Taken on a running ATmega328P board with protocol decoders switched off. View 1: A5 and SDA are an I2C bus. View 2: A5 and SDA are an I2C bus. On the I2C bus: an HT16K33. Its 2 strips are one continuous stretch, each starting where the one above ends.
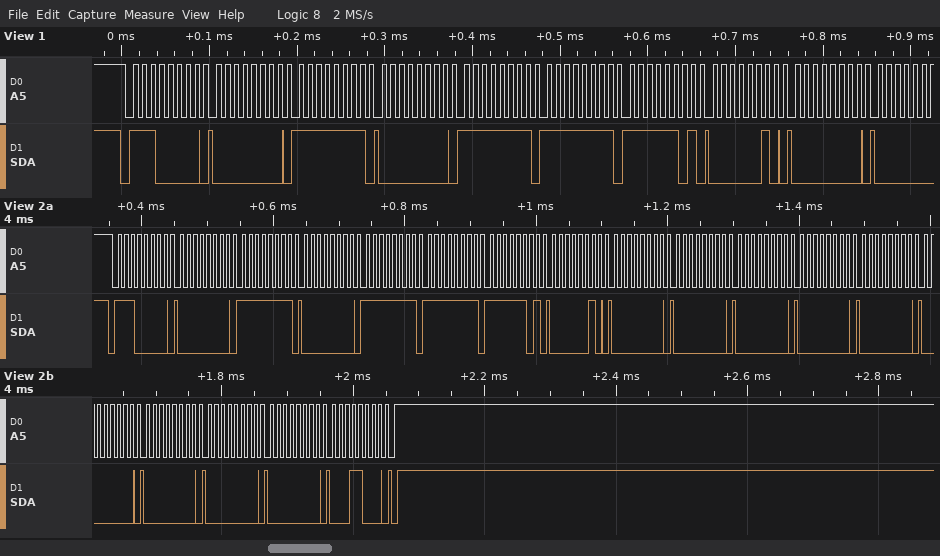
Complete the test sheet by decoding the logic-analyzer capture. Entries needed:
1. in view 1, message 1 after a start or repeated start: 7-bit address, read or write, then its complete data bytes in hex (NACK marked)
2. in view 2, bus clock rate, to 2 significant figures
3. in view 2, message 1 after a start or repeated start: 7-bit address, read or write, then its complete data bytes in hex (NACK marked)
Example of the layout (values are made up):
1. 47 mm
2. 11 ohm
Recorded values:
1. 0x70 write: 00 FF 00 FF FF FD 02 00
2. 100 kHz
3. 0x70 write: 00 FF 00 FF FF FD 02 00 00 00 00 00 00 00 00 00 18
